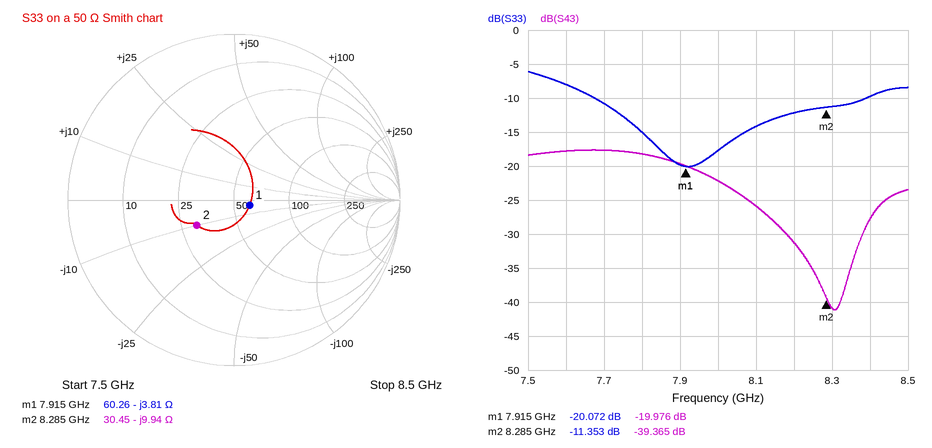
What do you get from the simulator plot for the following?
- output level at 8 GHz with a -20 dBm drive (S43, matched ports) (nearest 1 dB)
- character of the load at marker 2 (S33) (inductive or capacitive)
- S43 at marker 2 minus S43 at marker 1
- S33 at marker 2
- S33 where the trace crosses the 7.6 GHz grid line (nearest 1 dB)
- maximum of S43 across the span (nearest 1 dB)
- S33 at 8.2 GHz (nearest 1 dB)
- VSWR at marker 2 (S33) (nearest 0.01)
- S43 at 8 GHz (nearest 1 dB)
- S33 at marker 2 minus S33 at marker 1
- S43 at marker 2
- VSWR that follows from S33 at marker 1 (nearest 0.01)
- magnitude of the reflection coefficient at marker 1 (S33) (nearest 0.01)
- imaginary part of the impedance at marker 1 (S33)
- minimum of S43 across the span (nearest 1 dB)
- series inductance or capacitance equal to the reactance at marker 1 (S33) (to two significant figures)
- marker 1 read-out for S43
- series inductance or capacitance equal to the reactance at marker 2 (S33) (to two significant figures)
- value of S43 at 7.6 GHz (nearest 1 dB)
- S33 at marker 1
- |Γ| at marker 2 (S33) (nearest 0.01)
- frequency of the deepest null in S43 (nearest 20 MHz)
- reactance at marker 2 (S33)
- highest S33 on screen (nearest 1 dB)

-42 dBm
capacitive
-19.389 dB
-11.353 dB
-8 dB
-18 dB
-12 dB
1.74
-22 dB
8.719 dB
-39.365 dB
1.22
0.10
-3.81 Ω
-41 dB
5.3 pF
-19.976 dB
1.9 pF
-18 dB
-20.072 dB
0.27
8.30 GHz
-9.94 Ω
-6 dB
